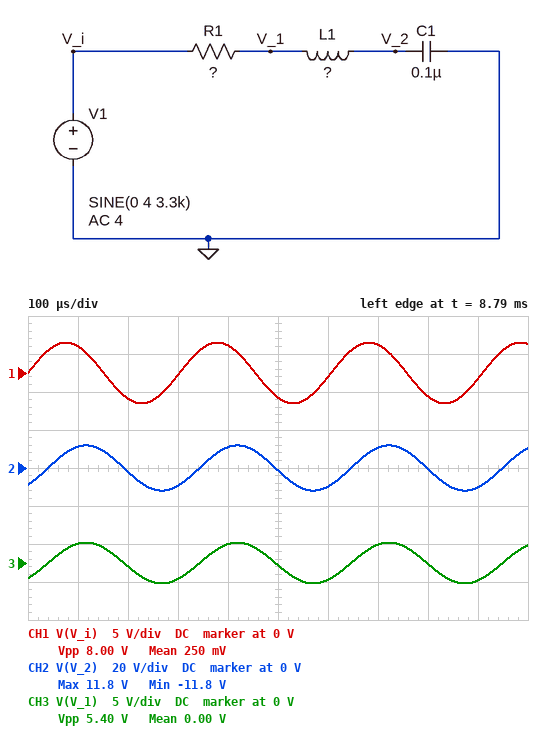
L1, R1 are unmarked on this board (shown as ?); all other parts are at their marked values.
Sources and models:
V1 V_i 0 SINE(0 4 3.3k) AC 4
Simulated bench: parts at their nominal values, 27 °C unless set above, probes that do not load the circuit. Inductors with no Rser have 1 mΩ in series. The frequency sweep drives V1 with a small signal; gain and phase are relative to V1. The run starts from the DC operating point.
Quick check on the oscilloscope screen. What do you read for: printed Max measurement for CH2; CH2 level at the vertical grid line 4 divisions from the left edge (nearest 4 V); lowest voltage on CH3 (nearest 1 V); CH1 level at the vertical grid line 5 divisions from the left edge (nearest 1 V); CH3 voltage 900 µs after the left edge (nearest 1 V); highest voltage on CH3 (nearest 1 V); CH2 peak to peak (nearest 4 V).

11.8 V
12 V
-3 V
-3 V
-2 V
3 V
24 V
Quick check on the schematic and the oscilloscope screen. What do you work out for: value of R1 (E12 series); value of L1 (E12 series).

120 Ω
18 mH
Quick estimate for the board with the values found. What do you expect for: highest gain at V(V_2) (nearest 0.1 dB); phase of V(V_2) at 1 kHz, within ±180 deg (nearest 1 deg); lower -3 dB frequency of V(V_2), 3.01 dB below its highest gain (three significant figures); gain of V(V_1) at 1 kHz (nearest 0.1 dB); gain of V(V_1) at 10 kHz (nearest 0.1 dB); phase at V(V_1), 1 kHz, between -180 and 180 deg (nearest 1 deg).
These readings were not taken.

11.1 dB
-5 deg
3.09 kHz
0 dB
-0.1 dB
-5 deg
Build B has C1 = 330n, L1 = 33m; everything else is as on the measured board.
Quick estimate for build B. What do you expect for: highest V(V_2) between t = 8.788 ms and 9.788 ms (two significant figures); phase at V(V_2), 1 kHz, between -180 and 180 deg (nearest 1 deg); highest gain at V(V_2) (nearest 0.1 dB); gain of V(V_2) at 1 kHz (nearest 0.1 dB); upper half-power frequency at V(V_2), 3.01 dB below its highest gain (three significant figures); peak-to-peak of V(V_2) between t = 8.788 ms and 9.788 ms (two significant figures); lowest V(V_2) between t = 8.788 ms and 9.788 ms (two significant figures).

1.1 V
-24 deg
8.6 dB
4.1 dB
1.74 kHz
2.1 V
-1.1 V
